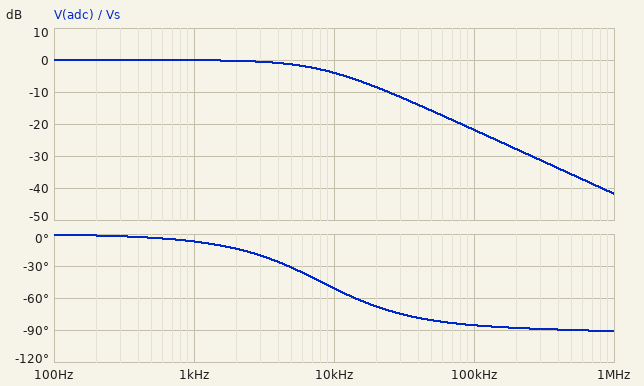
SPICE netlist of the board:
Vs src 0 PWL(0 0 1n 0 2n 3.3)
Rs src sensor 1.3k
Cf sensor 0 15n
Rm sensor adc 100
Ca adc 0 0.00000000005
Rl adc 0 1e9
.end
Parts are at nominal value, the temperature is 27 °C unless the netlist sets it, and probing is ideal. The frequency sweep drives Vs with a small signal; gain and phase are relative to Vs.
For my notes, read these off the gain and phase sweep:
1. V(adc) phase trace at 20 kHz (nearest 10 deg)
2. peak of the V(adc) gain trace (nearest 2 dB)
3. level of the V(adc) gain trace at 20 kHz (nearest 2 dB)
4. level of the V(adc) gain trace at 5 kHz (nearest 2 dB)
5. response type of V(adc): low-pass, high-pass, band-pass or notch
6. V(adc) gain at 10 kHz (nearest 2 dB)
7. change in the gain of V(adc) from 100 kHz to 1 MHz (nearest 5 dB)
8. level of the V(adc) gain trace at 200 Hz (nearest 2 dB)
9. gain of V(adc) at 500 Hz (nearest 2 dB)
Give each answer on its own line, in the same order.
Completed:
-70 deg
0 dB
-8 dB
-2 dB
low-pass
-4 dB
-20 dB
0 dB
0 dB
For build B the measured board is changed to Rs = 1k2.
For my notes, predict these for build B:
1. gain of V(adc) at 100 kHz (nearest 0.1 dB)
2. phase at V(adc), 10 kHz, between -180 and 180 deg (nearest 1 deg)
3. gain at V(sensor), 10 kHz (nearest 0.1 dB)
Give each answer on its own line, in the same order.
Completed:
-21.1 dB
-49 deg
-3.6 dB
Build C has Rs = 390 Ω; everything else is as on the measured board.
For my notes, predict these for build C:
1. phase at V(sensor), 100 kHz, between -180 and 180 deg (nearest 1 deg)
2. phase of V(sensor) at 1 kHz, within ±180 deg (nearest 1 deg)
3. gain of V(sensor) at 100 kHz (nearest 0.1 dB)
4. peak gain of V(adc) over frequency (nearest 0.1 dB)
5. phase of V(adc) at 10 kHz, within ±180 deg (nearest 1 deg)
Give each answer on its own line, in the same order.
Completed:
-75 deg
-2 deg
-11.6 dB
0 dB
-20 deg
